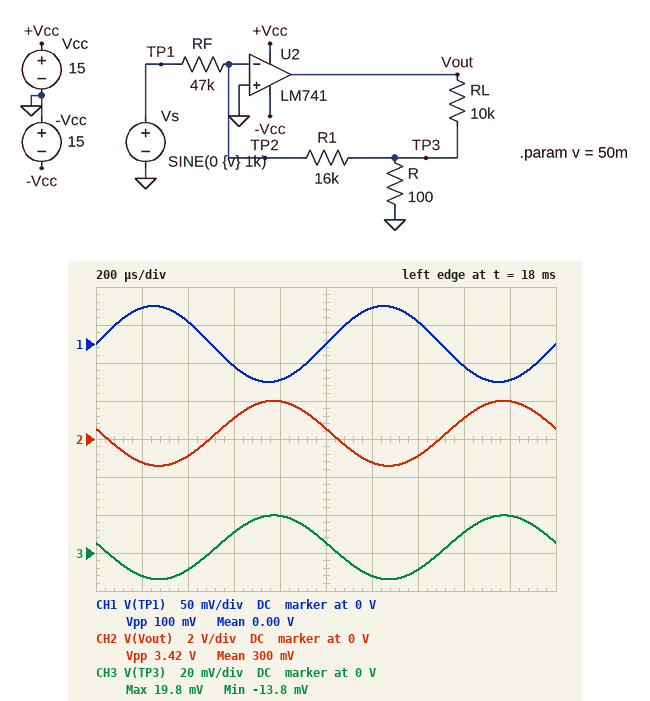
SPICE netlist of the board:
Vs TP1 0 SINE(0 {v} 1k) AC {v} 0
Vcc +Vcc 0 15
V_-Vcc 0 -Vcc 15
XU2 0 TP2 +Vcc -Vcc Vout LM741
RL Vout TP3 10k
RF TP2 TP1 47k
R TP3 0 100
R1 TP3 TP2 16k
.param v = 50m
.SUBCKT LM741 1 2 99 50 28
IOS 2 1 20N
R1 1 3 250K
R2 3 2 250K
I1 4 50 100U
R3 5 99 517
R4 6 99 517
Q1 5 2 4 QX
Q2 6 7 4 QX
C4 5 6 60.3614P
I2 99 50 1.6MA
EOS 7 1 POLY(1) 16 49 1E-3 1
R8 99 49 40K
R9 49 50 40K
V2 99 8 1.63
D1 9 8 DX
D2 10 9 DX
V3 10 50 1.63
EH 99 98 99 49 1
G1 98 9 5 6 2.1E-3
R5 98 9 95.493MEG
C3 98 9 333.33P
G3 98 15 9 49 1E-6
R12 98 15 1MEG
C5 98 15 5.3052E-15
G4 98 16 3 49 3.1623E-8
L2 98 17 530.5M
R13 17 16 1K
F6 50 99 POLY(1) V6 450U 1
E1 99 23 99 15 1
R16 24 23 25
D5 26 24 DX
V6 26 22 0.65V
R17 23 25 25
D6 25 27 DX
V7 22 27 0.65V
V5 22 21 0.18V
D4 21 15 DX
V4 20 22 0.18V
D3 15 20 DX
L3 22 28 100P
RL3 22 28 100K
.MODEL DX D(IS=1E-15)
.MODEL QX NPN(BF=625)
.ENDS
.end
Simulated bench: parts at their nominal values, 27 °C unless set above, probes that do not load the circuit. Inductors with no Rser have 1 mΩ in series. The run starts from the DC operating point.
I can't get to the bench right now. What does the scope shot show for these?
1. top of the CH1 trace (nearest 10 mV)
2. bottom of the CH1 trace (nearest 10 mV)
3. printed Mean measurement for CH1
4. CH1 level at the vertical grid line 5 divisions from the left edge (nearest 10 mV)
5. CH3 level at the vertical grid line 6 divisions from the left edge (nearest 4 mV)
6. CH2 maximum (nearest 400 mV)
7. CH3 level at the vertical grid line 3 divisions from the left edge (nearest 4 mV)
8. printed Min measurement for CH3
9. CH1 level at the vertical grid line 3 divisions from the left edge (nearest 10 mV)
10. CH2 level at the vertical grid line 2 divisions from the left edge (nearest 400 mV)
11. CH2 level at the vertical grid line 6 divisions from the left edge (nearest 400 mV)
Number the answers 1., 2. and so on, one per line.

1. 50 mV
2. -50 mV
3. 0.00 V
4. 0 V
5. -12 mV
6. 2.0 V
7. 12 mV
8. -13.8 mV
9. -30 mV
10. -800 mV
11. -1.2 V
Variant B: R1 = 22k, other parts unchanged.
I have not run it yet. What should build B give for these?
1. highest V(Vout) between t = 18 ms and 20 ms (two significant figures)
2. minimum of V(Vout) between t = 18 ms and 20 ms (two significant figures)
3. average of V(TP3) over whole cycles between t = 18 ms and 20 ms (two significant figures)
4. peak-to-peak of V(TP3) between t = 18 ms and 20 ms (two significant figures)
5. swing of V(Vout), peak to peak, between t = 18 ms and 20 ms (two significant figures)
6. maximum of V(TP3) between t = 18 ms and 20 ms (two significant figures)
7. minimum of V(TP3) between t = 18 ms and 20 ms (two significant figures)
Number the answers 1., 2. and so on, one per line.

1. 2.7 V
2. -2.0 V
3. 3.7 mV
4. 46 mV
5. 4.7 V
6. 27 mV
7. -19 mV
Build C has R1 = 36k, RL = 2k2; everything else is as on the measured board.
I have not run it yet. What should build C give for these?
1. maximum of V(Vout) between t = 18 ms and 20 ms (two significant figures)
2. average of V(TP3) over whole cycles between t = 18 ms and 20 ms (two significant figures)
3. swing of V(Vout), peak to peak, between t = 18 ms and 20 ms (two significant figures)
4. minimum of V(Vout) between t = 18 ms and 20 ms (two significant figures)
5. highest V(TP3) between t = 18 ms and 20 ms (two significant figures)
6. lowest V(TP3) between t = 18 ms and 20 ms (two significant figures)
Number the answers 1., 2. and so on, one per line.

1. 1.0 V
2. 5.4 mV
3. 1.8 V
4. -760 mV
5. 44 mV
6. -33 mV
